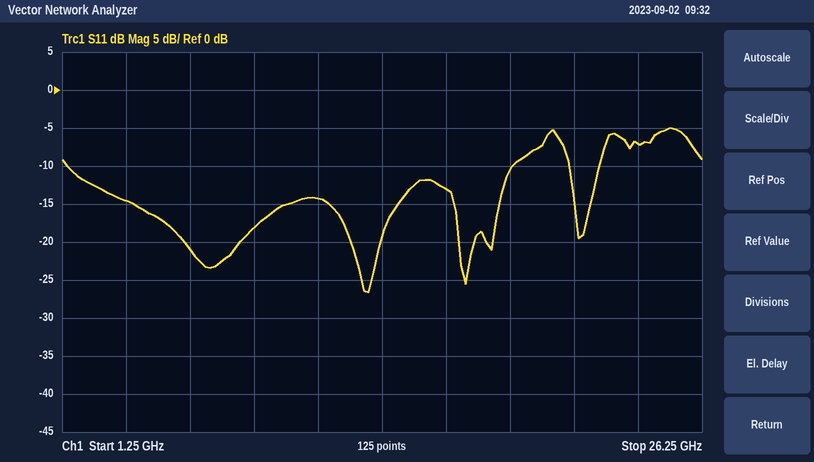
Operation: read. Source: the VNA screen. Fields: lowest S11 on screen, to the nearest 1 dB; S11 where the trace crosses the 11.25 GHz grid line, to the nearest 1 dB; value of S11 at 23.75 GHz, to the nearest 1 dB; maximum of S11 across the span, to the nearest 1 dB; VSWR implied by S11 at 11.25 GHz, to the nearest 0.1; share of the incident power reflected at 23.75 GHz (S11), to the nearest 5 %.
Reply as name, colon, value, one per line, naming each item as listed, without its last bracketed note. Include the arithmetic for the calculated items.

lowest S11 on screen, to the nearest 1 dB: -27 dB
S11 where the trace crosses the 11.25 GHz grid line, to the nearest 1 dB: -14 dB
value of S11 at 23.75 GHz, to the nearest 1 dB: -7 dB
maximum of S11 across the span, to the nearest 1 dB: -5 dB
VSWR implied by S11 at 11.25 GHz, to the nearest 0.1: |Γ| = 10^(-14/20) = 0.1995; VSWR = (1 + 0.1995)/(1 − 0.1995) ≈ 1.5
share of the incident power reflected at 23.75 GHz (S11), to the nearest 5 %: 10^(-7/10) ≈ 20 %
